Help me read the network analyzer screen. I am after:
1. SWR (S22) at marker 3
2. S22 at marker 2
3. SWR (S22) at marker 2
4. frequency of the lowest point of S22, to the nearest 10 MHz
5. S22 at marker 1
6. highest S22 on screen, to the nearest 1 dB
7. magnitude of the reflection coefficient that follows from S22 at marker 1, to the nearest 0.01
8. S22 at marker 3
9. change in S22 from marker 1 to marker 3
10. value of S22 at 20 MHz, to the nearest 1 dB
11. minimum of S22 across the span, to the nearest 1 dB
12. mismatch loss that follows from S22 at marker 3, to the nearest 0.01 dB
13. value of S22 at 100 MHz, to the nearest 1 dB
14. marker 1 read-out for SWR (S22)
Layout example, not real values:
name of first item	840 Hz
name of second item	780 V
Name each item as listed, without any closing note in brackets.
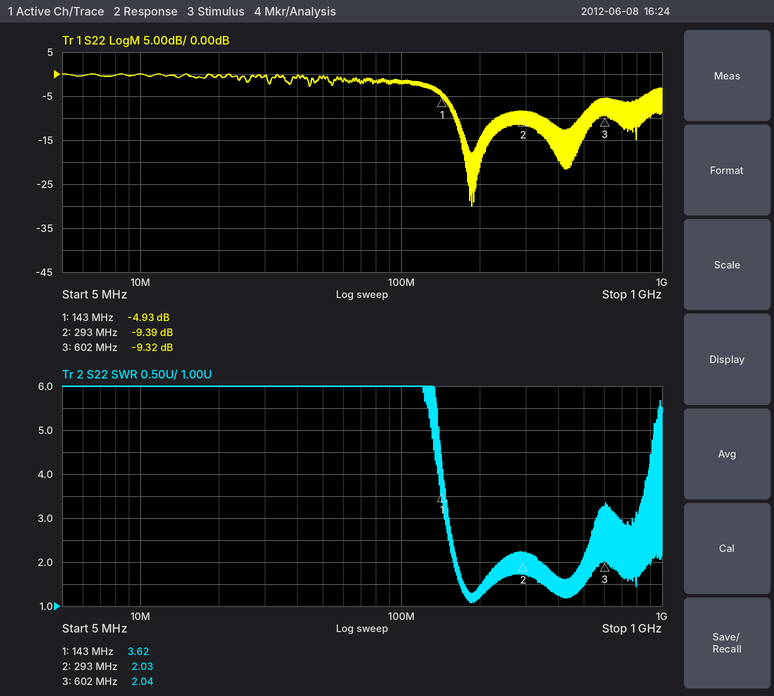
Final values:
SWR (S22) at marker 3	2.04
S22 at marker 2	-9.39 dB
SWR (S22) at marker 2	2.03
frequency of the lowest point of S22, to the nearest 10 MHz	190 MHz
S22 at marker 1	-4.93 dB
highest S22 on screen, to the nearest 1 dB	0 dB
magnitude of the reflection coefficient that follows from S22 at marker 1, to the nearest 0.01	0.57
S22 at marker 3	-9.32 dB
change in S22 from marker 1 to marker 3	-4.39 dB
value of S22 at 20 MHz, to the nearest 1 dB	0 dB
minimum of S22 across the span, to the nearest 1 dB	-30 dB
mismatch loss that follows from S22 at marker 3, to the nearest 0.01 dB	0.54 dB
value of S22 at 100 MHz, to the nearest 1 dB	-2 dB
marker 1 read-out for SWR	3.62
